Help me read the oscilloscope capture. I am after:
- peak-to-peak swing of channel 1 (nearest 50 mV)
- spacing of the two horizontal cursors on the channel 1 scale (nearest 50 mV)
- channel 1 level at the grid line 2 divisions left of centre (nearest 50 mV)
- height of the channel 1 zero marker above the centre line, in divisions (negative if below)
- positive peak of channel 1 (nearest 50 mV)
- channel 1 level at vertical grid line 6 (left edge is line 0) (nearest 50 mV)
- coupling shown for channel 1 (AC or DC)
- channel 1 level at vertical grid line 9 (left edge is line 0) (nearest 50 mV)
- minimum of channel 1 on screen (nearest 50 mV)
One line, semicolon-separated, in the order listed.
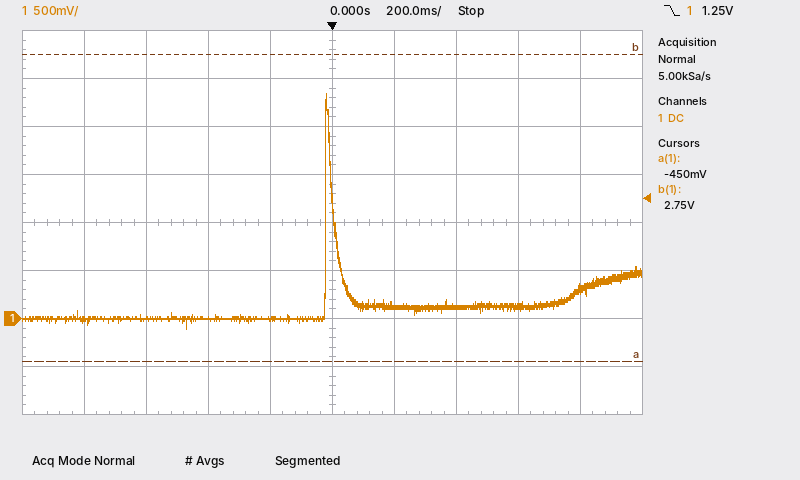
2.45 V; 3.20 V; 0 mV; -2.0 div; 2.35 V; 150 mV; DC; 300 mV; -100 mV
